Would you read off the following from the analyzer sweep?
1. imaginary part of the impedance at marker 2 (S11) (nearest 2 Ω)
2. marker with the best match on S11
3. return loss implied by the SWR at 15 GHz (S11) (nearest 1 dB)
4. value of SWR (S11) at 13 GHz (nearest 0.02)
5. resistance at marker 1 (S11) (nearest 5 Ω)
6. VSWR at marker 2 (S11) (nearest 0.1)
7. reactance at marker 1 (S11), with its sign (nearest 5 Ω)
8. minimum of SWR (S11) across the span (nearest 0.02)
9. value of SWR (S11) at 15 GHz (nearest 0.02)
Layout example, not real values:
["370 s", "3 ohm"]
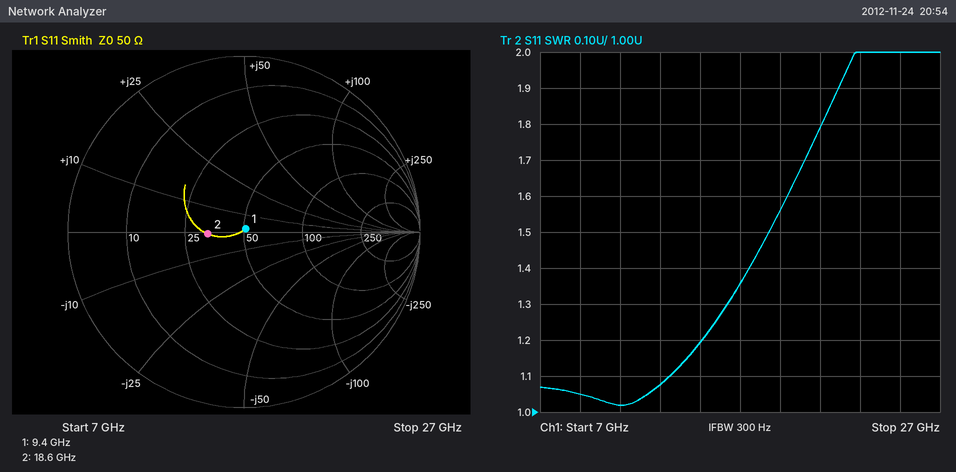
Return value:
["0 Ω", "marker 1", "21 dB", "1.08", "50 Ω", "1.5", "0 Ω", "1.02", "1.20"]
